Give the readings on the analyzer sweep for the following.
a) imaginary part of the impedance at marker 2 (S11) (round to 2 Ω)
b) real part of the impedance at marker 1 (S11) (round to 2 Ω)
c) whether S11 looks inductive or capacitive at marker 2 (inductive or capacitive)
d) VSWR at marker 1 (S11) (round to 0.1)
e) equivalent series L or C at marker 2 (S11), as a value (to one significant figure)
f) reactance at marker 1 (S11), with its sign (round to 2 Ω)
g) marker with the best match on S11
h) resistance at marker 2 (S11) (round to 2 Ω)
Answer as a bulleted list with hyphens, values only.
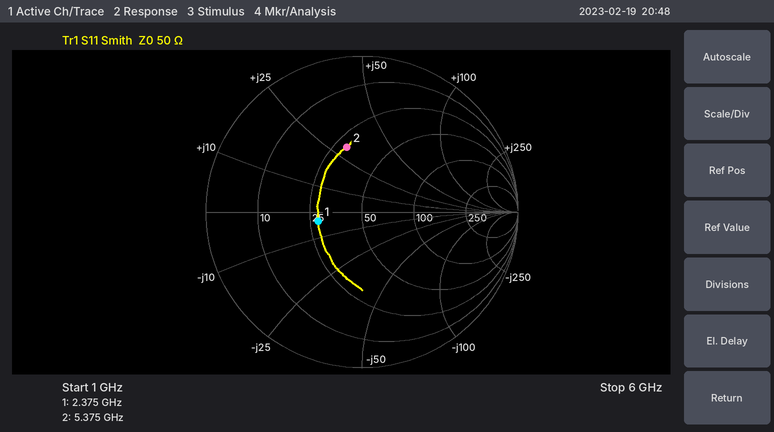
- +30 Ω
- 28 Ω
- inductive
- 1.8
- 900 pH
- -4 Ω
- marker 1
- 30 Ω
